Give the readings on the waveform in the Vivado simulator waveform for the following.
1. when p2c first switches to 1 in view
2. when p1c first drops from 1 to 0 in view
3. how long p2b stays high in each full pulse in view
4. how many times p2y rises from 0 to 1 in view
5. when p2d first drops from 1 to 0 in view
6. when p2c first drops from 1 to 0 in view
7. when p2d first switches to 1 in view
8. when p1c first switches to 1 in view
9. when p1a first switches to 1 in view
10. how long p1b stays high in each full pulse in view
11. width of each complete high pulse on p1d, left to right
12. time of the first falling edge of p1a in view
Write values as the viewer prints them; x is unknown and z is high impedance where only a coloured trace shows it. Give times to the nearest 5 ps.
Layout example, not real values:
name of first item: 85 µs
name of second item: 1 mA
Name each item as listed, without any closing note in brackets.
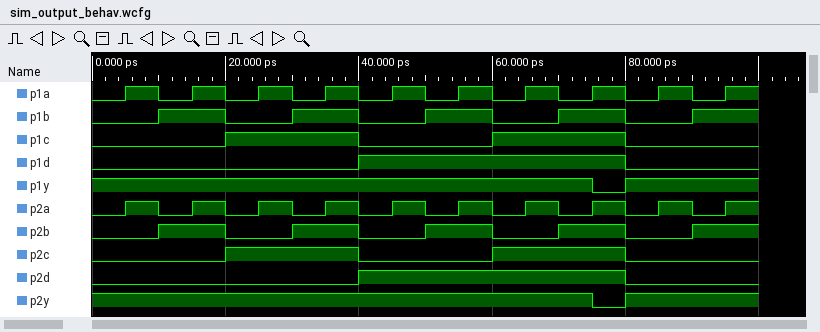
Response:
when p2c first switches to 1 in view: 20 ps
when p1c first drops from 1 to 0 in view: 40 ps
how long p2b stays high in each full pulse in view: 10 ps, 10 ps, 10 ps, 10 ps
how many times p2y rises from 0 to 1 in view: 1
when p2d first drops from 1 to 0 in view: 80 ps
when p2c first drops from 1 to 0 in view: 40 ps
when p2d first switches to 1 in view: 40 ps
when p1c first switches to 1 in view: 20 ps
when p1a first switches to 1 in view: 5 ps
how long p1b stays high in each full pulse in view: 10 ps, 10 ps, 10 ps, 10 ps
width of each complete high pulse on p1d, left to right: 40 ps
time of the first falling edge of p1a in view: 10 ps
